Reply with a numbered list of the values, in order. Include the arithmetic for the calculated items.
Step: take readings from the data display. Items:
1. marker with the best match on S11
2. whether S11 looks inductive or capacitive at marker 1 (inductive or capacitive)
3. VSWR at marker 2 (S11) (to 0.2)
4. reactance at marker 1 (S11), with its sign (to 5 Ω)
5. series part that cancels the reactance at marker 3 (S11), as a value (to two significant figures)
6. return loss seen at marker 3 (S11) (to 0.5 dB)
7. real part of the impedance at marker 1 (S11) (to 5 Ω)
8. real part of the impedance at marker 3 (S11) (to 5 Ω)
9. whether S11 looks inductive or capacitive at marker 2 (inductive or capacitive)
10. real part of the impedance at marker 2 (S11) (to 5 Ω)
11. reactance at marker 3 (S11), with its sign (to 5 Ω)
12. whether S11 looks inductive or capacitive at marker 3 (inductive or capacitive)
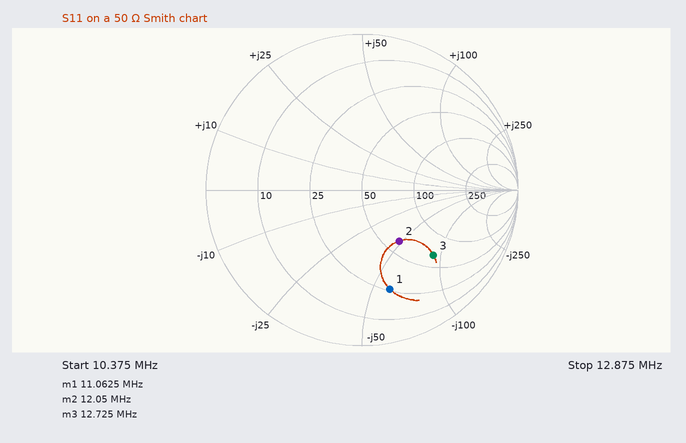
1. marker 2
2. capacitive
3. 2.4
4. -60 Ω
5. L = 90 Ω/(2π × 12.725 MHz) ≈ 1.1 µH
6. 4.0 dB
7. 25 Ω
8. 65 Ω
9. capacitive
10. 60 Ω
11. -90 Ω
12. capacitive
